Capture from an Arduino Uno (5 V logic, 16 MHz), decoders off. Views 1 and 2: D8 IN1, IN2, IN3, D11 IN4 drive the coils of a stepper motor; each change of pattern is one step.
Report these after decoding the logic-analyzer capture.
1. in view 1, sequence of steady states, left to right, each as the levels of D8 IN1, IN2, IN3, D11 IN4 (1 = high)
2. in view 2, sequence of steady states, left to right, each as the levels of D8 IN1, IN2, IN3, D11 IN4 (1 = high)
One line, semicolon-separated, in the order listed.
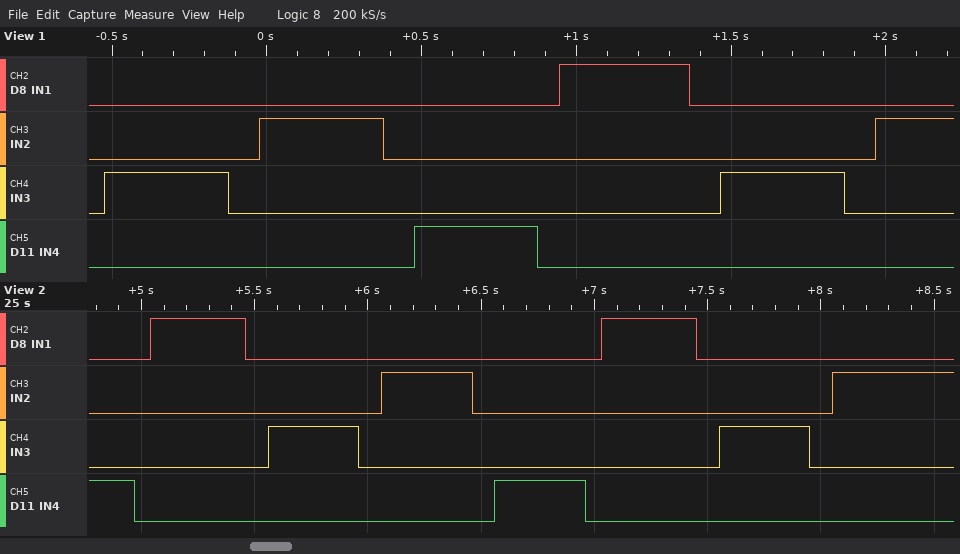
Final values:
0000 0010 0000 0100 0000 0001 0000 1000 0000 0010 0000 0100; 0001 0000 1000 0000 0010 0000 0100 0000 0001 0000 1000 0000 0010 0000 0100
